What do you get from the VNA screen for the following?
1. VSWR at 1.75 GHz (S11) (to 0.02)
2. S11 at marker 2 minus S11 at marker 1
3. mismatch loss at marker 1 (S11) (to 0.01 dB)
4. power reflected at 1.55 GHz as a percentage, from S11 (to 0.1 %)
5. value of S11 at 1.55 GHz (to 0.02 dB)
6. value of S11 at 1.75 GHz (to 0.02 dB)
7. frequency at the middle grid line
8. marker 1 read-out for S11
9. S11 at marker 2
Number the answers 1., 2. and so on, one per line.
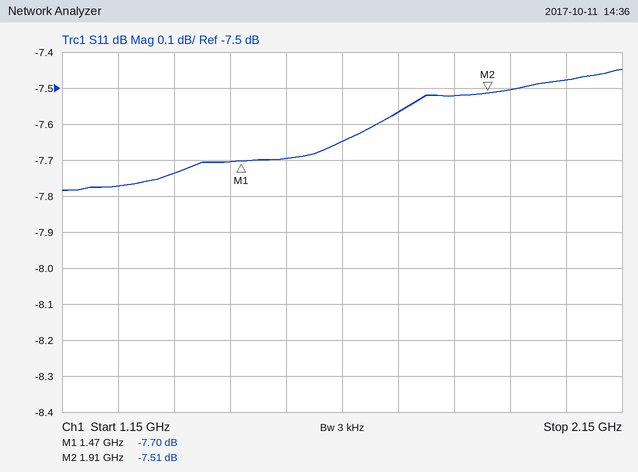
1. 2.44
2. 0.19 dB
3. 0.81 dB
4. 17.0 %
5. -7.70 dB
6. -7.56 dB
7. 1.65 GHz
8. -7.70 dB
9. -7.51 dB
